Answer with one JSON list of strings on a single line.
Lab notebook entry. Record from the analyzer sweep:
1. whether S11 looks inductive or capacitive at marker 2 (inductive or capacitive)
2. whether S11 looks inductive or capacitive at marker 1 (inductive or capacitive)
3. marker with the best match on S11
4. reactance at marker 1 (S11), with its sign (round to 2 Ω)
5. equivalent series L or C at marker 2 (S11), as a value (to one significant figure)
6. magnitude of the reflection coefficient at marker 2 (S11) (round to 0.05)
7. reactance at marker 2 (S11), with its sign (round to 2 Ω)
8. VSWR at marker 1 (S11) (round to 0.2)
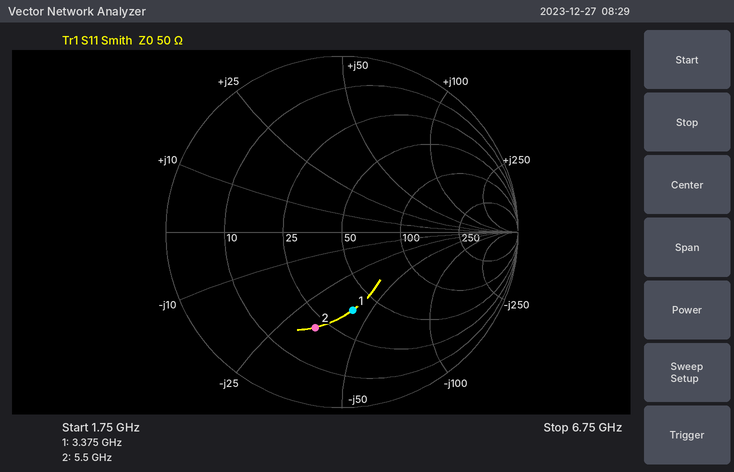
["capacitive", "capacitive", "marker 1", "-42 Ω", "900 fF", "0.55", "-34 Ω", "2.6"]
